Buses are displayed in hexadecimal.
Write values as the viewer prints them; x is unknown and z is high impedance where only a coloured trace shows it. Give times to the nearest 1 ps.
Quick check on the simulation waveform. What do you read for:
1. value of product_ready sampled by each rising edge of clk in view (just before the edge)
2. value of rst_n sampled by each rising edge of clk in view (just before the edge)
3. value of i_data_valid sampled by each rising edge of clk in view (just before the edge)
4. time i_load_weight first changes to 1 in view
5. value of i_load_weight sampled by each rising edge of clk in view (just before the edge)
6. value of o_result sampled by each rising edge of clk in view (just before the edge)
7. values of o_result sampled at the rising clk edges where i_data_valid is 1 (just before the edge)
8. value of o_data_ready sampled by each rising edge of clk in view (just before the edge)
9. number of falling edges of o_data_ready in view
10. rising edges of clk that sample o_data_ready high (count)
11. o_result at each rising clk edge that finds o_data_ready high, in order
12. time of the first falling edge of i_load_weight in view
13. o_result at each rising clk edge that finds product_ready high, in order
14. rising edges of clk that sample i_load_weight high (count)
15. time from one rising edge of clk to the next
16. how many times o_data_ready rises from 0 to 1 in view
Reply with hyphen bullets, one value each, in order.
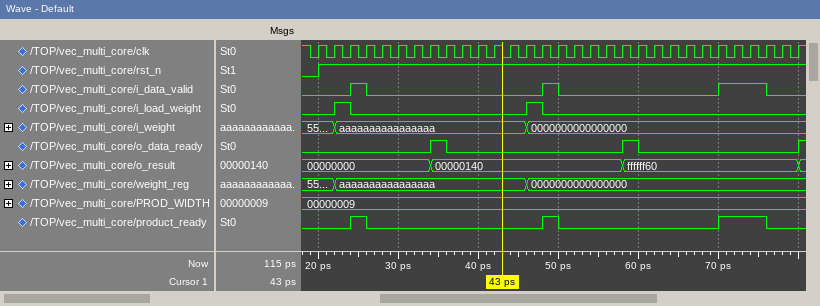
- 0 0 0 1 0 0 0 0 0 0 0 0 0 0 0 1 0 0 0 0 0 0 0 0 0 0 1 1 1 0 0
- 0 1 1 1 1 1 1 1 1 1 1 1 1 1 1 1 1 1 1 1 1 1 1 1 1 1 1 1 1 1 1
- 0 0 0 1 0 0 0 0 0 0 0 0 0 0 0 1 0 0 0 0 0 0 0 0 0 0 1 1 1 0 0
- 22 ps
- 0 0 1 0 0 0 0 0 0 0 0 0 0 0 1 0 0 0 0 0 0 0 0 0 0 0 0 0 0 0 0
- 00000000, 00000000, 00000000, 00000000, 00000000, 00000000, 00000000, 00000000, 00000140, 00000140, 00000140, 00000140, 00000140, 00000140, 00000140, 00000140, 00000140, 00000140, 00000140, 00000140, ffffff60, ffffff60, ffffff60, ffffff60, ffffff60, ffffff60, ffffff60, ffffff60, ffffff60, ffffff60, ffffff60
- 00000000, 00000140, ffffff60, ffffff60, ffffff60
- 0 0 0 0 0 0 0 0 1 0 0 0 0 0 0 0 0 0 0 0 1 0 0 0 0 0 0 0 0 0 0
- 2
- 2
- 00000140, ffffff60
- 24 ps
- 00000000, 00000140, ffffff60, ffffff60, ffffff60
- 2
- 2 ps
- 3
